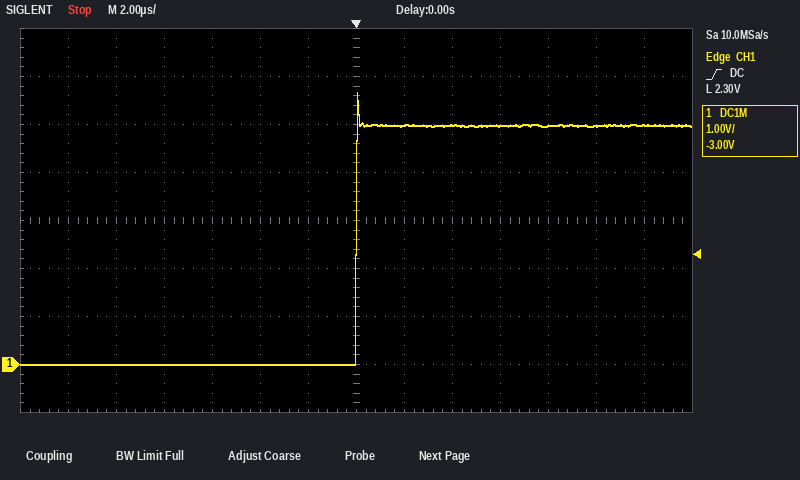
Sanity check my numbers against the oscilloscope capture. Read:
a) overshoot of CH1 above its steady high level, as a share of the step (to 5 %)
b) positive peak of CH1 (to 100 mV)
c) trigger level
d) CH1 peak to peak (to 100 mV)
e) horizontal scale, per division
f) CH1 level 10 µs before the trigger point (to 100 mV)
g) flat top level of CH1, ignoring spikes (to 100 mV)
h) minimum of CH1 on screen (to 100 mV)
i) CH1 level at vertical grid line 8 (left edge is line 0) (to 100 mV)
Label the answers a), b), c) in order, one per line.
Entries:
a) 15 %
b) 5.7 V
c) 2.30 V
d) 5.7 V
e) 2 µs
f) 0.0 V
g) 5.0 V
h) 0.0 V
i) 5.0 V
